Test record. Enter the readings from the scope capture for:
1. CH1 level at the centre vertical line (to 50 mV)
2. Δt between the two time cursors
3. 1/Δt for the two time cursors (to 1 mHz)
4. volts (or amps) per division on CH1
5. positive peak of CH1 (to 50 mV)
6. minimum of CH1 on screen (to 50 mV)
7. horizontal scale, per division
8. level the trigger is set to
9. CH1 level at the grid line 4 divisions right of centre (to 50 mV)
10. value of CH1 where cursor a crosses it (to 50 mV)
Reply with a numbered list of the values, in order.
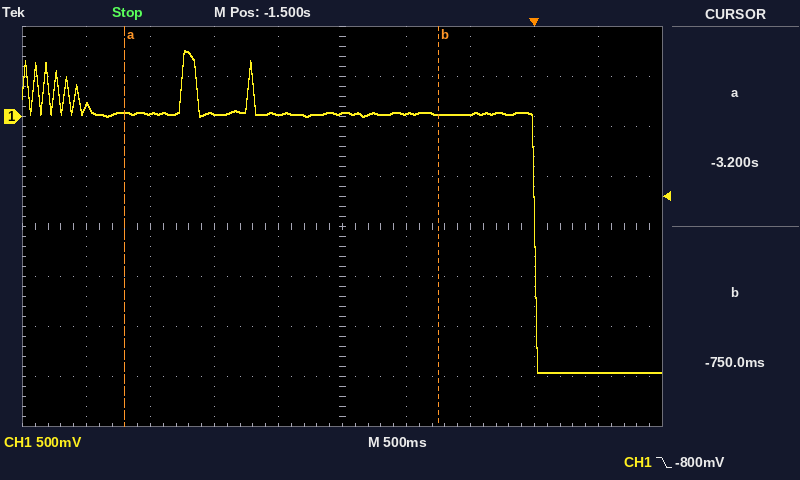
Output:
1. 50 mV
2. 2.45 s
3. 408 mHz
4. 500 mV
5. 650 mV
6. -2.55 V
7. 500 ms
8. -800 mV
9. -2.55 V
10. 50 mV
